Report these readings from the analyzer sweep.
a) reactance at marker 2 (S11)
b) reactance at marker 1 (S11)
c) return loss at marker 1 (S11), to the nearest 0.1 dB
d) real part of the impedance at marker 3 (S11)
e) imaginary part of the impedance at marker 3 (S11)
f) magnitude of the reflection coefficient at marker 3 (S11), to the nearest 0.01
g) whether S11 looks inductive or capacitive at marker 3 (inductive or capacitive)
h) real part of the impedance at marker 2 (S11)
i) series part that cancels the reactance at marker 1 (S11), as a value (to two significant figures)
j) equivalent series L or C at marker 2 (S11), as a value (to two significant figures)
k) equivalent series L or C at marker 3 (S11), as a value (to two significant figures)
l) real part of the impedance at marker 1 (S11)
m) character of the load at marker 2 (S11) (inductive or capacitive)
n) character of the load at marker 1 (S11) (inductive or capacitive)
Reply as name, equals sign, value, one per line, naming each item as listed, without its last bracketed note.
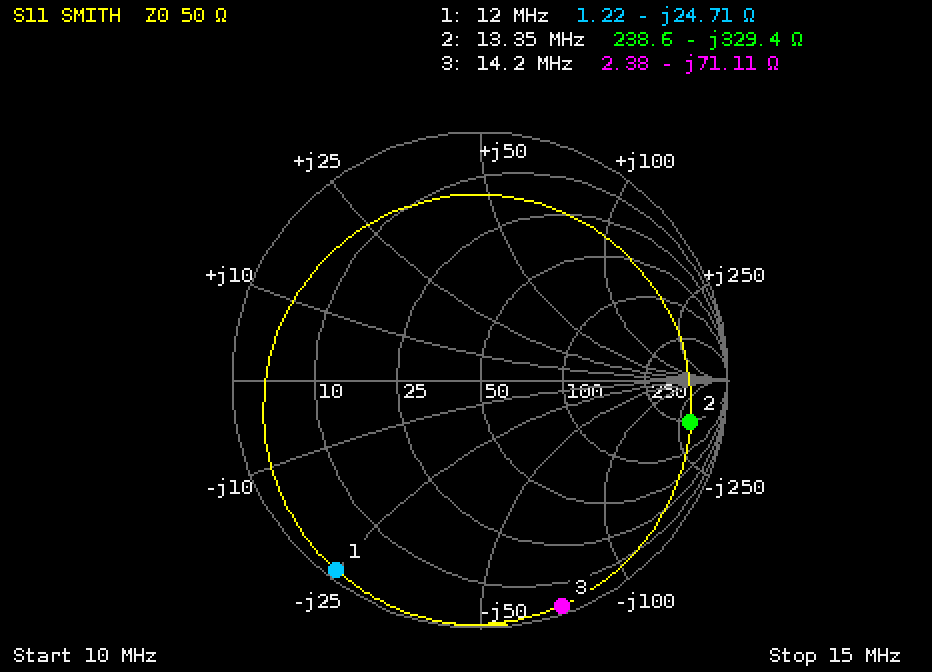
reactance at marker 2 = -329.4 Ω
reactance at marker 1 = -24.71 Ω
return loss at marker 1 (S11), to the nearest 0.1 dB = 0.3 dB
real part of the impedance at marker 3 = 2.38 Ω
imaginary part of the impedance at marker 3 = -71.11 Ω
magnitude of the reflection coefficient at marker 3 (S11), to the nearest 0.01 = 0.97
whether S11 looks inductive or capacitive at marker 3 = capacitive
real part of the impedance at marker 2 = 238.6 Ω
series part that cancels the reactance at marker 1 (S11), as a value = 330 nH
equivalent series L or C at marker 2 (S11), as a value = 36 pF
equivalent series L or C at marker 3 (S11), as a value = 160 pF
real part of the impedance at marker 1 = 1.22 Ω
character of the load at marker 2 (S11) = capacitive
character of the load at marker 1 (S11) = capacitive
